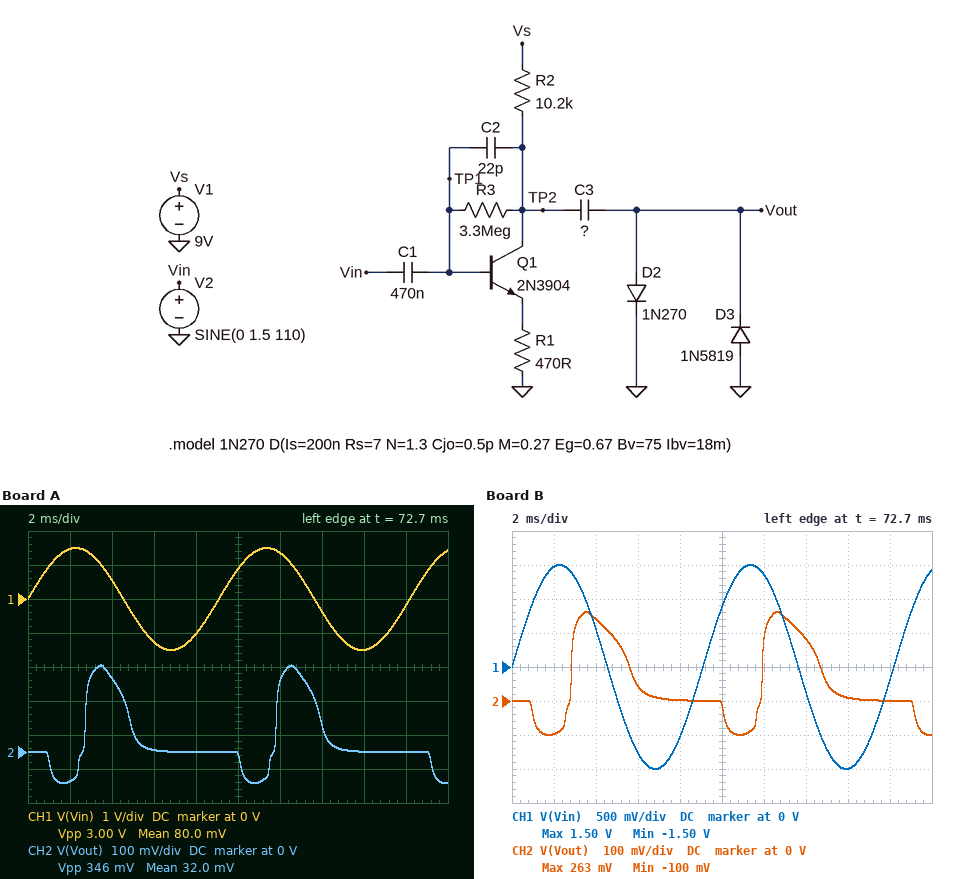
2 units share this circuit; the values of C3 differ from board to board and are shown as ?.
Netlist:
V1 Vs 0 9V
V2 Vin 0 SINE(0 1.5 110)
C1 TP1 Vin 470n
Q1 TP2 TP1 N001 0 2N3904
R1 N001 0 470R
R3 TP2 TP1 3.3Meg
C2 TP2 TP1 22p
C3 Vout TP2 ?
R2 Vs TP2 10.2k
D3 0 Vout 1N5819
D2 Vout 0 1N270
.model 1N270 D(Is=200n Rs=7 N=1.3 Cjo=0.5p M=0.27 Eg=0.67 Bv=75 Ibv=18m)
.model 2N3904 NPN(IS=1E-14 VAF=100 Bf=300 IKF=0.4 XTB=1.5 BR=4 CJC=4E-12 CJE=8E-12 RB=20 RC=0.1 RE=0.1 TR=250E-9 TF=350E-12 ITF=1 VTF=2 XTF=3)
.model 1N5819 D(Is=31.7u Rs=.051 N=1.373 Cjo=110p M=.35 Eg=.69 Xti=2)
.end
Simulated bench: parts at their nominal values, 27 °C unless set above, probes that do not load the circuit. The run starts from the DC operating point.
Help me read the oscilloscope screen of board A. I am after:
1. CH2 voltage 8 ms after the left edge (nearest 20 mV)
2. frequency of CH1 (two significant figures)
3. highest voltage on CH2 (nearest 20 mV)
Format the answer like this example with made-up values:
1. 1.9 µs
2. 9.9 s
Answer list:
1. 0 V
2. 110 Hz
3. 260 mV
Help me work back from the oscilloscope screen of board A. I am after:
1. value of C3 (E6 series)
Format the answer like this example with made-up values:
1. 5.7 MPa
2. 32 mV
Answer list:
1. 47 nF
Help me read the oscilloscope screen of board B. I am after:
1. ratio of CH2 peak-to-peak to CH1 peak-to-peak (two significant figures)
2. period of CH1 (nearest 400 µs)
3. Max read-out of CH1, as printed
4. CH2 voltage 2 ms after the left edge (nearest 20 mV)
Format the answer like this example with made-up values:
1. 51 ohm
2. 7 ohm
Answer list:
1. 0.12
2. 9.2 ms
3. 1.50 V
4. -100 mV
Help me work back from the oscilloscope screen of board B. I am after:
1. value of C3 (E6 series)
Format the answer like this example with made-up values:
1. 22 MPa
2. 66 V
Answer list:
1. 68 nF
